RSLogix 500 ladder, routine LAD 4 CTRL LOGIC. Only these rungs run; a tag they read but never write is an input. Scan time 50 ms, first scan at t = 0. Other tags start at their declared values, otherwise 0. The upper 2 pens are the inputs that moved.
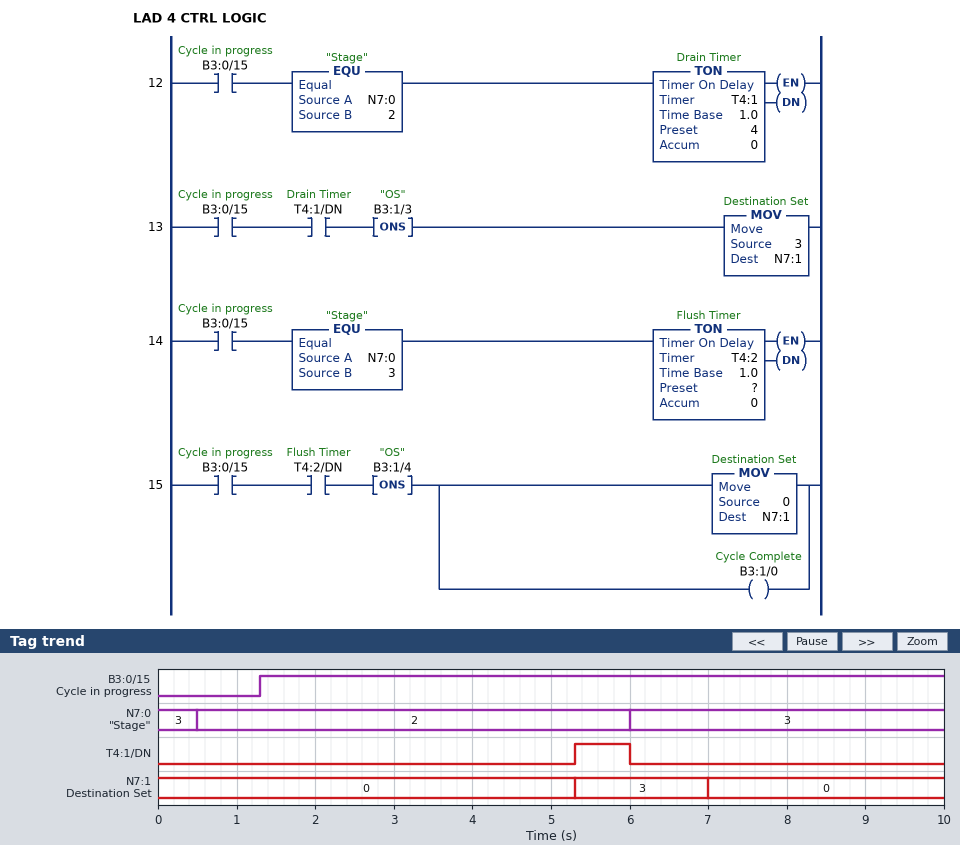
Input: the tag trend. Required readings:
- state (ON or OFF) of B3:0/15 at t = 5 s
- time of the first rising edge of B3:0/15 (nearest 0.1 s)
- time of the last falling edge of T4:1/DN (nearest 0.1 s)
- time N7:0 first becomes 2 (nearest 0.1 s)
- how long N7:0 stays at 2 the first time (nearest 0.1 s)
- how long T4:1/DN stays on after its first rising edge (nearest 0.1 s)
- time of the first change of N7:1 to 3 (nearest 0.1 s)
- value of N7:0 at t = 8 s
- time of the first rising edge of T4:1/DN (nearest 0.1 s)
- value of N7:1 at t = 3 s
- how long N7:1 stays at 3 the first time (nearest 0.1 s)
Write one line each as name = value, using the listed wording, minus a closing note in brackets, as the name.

state (ON or OFF) of B3:0/15 at t = 5 s = ON
time of the first rising edge of B3:0/15 = 1.3 s
time of the last falling edge of T4:1/DN = 6.0 s
time N7:0 first becomes 2 = 0.5 s
how long N7:0 stays at 2 the first time = 5.5 s
how long T4:1/DN stays on after its first rising edge = 0.7 s
time of the first change of N7:1 to 3 = 5.3 s
value of N7:0 at t = 8 s = 3
time of the first rising edge of T4:1/DN = 5.3 s
value of N7:1 at t = 3 s = 0
how long N7:1 stays at 3 the first time = 1.7 s
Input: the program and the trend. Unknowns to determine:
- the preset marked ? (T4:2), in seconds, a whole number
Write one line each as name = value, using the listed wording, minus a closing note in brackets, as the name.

the preset marked ? (T4:2), in seconds, a whole number = 1 s
